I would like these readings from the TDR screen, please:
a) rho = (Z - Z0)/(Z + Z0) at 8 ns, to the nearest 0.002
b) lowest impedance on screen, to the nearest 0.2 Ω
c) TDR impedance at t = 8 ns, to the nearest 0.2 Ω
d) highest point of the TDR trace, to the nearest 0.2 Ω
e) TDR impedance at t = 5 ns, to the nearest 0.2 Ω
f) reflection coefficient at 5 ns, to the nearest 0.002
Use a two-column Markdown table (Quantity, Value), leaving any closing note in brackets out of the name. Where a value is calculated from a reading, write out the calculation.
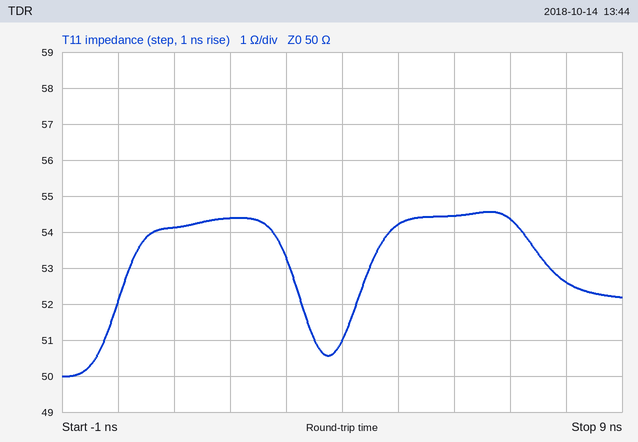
| Quantity | Value |
|---|---|
| rho = (Z - Z0)/(Z + Z0) at 8 ns, to the nearest 0.002 | (52.6 − 50)/(52.6 + 50) ≈ +0.0253, so +0.026 to the nearest 0.002 |
| lowest impedance on screen, to the nearest 0.2 Ω | 50.0 Ω |
| TDR impedance at t = 8 ns, to the nearest 0.2 Ω | 52.6 Ω |
| highest point of the TDR trace, to the nearest 0.2 Ω | 54.6 Ω |
| TDR impedance at t = 5 ns, to the nearest 0.2 Ω | 54.2 Ω |
| reflection coefficient at 5 ns, to the nearest 0.002 | (54.2 − 50)/(54.2 + 50) ≈ +0.040 |
